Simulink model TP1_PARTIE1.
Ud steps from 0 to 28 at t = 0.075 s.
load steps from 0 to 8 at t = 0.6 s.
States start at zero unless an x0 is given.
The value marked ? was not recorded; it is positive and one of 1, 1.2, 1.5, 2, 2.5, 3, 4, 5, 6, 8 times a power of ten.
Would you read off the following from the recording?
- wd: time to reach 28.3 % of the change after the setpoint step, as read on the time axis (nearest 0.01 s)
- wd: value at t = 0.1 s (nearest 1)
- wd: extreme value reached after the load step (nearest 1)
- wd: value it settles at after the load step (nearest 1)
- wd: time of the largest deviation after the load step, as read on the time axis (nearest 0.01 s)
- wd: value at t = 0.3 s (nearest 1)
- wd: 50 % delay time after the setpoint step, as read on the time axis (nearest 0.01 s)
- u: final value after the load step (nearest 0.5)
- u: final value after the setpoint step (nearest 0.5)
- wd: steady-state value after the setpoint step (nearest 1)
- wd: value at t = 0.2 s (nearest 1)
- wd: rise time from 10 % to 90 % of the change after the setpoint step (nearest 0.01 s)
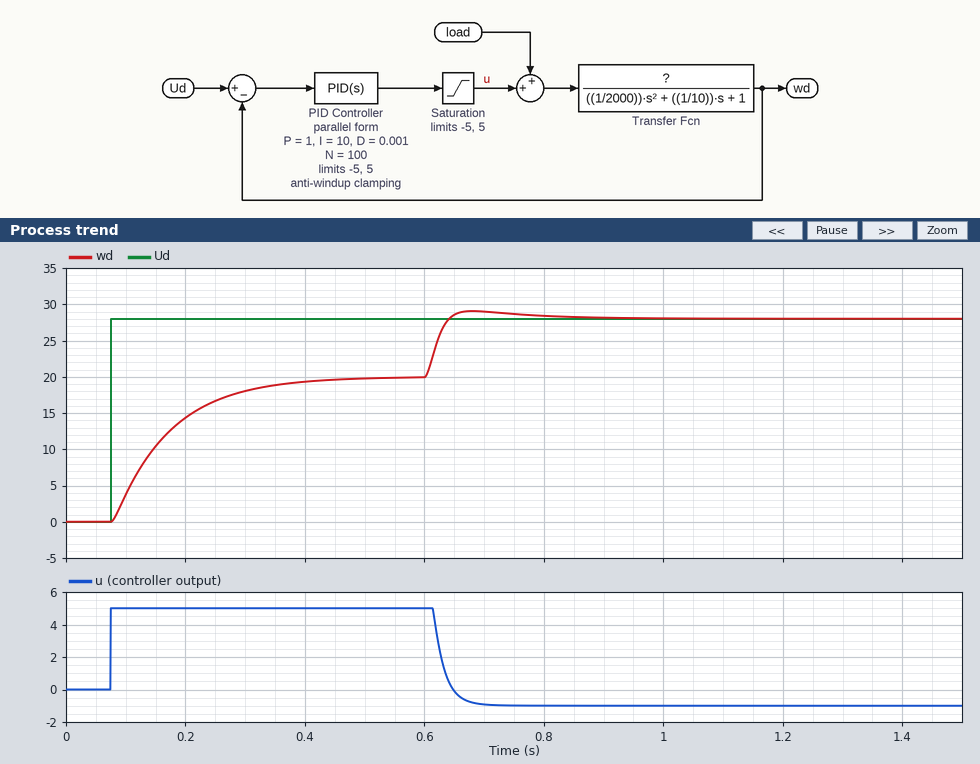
0.11 s
4
29
28
0.68 s
18
0.15 s
-1.0
5.0
20
14
0.21 s
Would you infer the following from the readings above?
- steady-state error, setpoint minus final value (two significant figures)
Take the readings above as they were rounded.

8.0
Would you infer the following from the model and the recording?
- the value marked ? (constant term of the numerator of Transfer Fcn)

4
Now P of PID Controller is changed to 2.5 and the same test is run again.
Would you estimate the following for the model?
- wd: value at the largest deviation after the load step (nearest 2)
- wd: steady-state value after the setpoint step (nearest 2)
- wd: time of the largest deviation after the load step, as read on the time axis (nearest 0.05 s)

28
20
0.65 s
